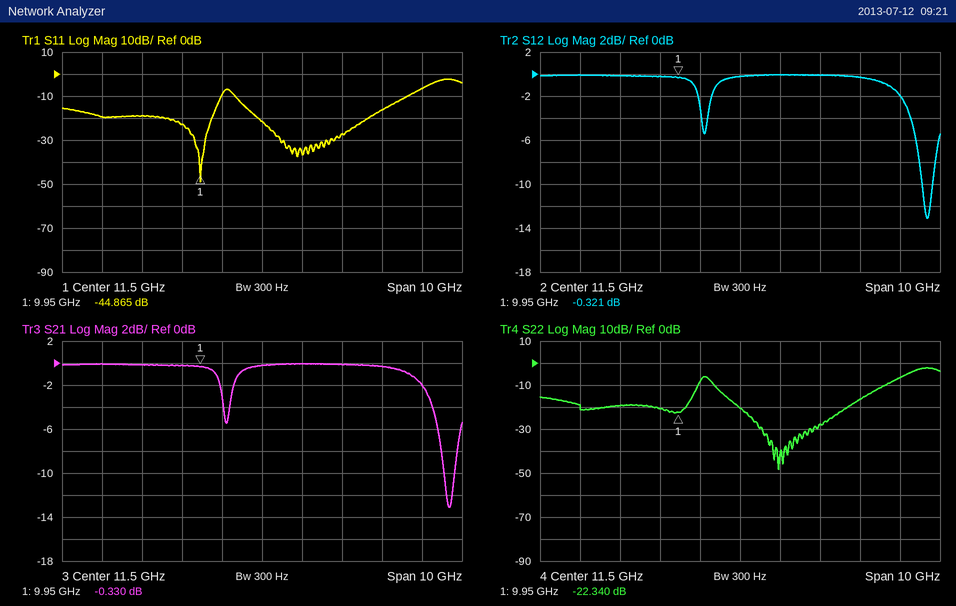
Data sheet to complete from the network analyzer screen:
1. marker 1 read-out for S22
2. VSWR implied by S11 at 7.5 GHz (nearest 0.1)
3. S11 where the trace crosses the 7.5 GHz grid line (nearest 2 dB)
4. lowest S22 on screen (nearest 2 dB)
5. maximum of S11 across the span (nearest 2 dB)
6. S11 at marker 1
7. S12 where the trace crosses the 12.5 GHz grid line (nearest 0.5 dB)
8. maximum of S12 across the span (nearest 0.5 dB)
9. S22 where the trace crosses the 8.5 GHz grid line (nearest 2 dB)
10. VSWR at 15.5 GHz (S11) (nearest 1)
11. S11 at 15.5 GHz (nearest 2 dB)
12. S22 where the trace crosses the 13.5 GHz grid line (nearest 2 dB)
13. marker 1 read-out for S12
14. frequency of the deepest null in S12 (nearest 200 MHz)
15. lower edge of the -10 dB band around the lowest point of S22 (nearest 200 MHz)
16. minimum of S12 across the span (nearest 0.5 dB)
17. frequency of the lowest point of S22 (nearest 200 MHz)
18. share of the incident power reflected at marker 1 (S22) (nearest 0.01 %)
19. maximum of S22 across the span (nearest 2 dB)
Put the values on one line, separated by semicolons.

-22.340 dB; 1.2; -20 dB; -48 dB; -2 dB; -44.865 dB; 0.0 dB; 0.0 dB; -20 dB; 3; -6 dB; -28 dB; -0.321 dB; 16.2 GHz; 10.8 GHz; -13.0 dB; 12.4 GHz; 0.58 %; -2 dB
